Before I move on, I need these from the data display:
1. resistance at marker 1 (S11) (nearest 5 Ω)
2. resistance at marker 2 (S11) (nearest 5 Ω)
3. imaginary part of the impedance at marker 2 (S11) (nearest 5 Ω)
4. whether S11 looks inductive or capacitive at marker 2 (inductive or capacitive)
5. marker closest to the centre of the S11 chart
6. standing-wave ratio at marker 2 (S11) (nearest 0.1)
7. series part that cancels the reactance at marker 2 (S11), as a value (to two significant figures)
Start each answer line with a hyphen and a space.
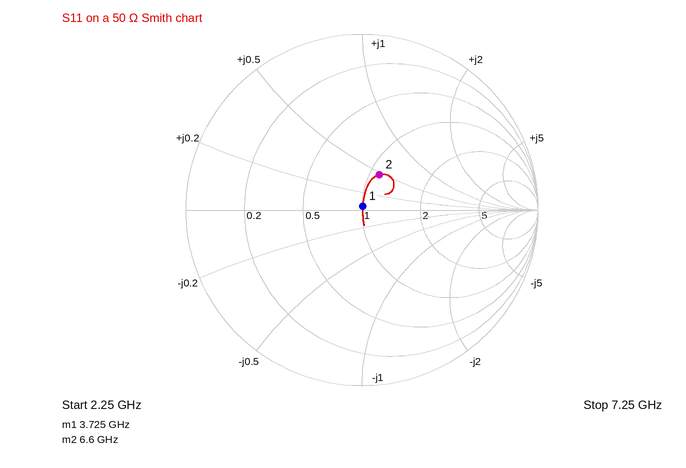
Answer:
- 50 Ω
- 55 Ω
- +25 Ω
- inductive
- marker 1
- 1.6
- 1.0 pF
